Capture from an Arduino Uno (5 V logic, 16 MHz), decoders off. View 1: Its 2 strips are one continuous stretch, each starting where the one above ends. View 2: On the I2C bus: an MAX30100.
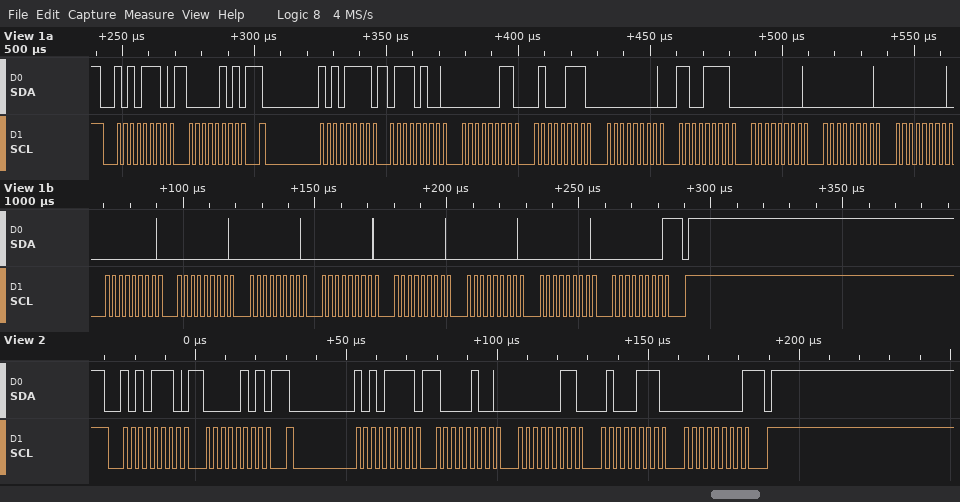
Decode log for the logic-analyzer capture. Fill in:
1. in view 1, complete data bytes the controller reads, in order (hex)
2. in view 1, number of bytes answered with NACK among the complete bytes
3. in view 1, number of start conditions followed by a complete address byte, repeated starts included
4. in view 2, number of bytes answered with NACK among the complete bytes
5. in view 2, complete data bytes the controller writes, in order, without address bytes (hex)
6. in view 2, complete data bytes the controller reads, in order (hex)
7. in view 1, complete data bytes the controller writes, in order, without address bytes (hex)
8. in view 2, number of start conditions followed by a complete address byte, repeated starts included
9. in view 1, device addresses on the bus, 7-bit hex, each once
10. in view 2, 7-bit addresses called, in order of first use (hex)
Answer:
74 03 47 00 CF 00 00 00 00 00 00 00 00 00 00 00
1
2
1
05
84 03 47 00
05
2
0x57
0x57
